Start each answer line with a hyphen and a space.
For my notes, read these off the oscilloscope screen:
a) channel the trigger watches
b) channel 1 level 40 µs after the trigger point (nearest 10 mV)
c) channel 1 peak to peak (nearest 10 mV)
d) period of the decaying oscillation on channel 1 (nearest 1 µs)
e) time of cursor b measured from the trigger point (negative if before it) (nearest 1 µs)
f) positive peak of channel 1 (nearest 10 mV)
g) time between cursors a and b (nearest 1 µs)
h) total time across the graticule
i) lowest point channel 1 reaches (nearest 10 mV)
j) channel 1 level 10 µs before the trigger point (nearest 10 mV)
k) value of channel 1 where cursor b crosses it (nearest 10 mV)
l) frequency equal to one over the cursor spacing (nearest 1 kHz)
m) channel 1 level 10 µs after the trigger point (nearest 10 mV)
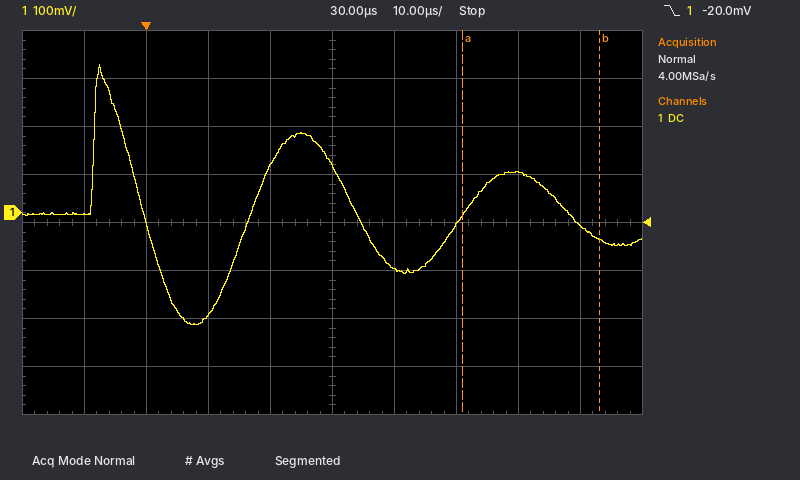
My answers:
- channel 1
- -120 mV
- 540 mV
- 34 µs
- +73 µs
- 310 mV
- 22 µs
- 100 µs
- -230 mV
- 0 mV
- -60 mV
- 45 kHz
- -210 mV
